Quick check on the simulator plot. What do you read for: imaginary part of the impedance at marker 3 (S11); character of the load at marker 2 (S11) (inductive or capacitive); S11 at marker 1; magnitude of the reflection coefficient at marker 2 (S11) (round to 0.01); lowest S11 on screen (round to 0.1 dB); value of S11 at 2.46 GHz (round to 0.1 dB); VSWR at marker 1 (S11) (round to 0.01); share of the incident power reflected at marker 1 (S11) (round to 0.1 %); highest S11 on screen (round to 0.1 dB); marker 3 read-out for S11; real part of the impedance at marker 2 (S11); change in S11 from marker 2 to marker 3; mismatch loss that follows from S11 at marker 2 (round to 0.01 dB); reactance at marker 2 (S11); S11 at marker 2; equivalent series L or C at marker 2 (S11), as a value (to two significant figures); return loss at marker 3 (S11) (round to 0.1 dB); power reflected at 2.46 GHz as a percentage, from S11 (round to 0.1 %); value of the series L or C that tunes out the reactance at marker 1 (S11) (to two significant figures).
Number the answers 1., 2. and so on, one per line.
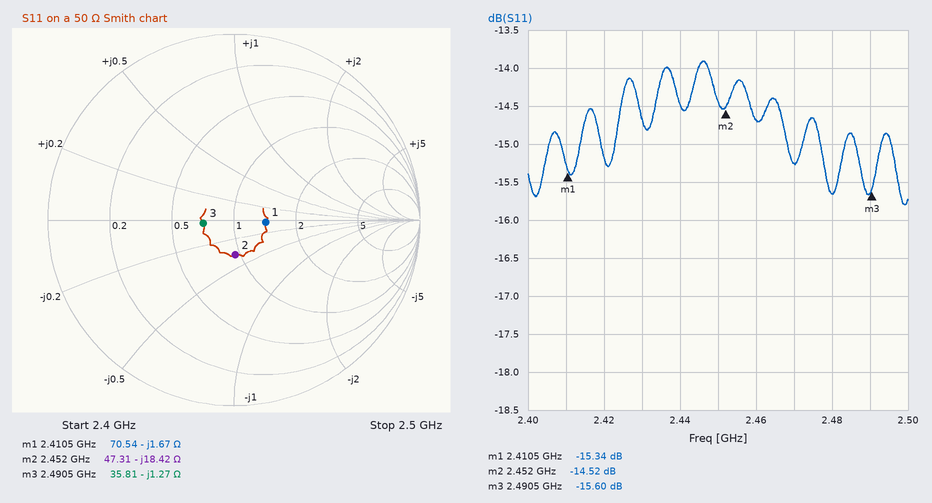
1. -1.27 Ω
2. capacitive
3. -15.34 dB
4. 0.19
5. -15.8 dB
6. -14.7 dB
7. 1.41
8. 2.9 %
9. -13.9 dB
10. -15.60 dB
11. 47.31 Ω
12. -1.08 dB
13. 0.16 dB
14. -18.42 Ω
15. -14.52 dB
16. 3.5 pF
17. 15.6 dB
18. 3.4 %
19. 110 pH
